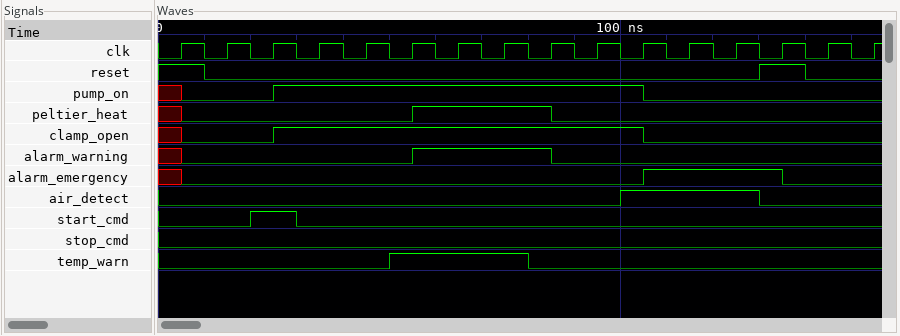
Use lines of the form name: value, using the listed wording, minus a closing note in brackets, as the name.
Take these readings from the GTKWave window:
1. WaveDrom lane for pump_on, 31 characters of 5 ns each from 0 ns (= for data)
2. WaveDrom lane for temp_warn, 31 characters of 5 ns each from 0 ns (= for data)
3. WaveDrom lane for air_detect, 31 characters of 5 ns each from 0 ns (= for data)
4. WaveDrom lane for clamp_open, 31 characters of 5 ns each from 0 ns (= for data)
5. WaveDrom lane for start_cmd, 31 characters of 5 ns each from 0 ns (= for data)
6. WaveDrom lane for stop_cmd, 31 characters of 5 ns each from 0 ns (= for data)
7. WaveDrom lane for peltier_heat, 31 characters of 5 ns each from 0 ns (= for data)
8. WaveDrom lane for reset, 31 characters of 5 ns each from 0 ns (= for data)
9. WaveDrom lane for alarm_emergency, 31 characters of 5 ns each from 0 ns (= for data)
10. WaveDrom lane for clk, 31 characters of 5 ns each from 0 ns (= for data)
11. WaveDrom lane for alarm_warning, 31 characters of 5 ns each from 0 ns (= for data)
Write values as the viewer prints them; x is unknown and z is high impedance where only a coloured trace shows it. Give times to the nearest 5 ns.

WaveDrom lane for pump_on, 31 characters of 5 ns each from 0 ns: {name: 'pump_on', wave: 'x0...1...............0.........'}
WaveDrom lane for temp_warn, 31 characters of 5 ns each from 0 ns: {name: 'temp_warn', wave: '0.........1.....0..............'}
WaveDrom lane for air_detect, 31 characters of 5 ns each from 0 ns: {name: 'air_detect', wave: '0...................1.....0....'}
WaveDrom lane for clamp_open, 31 characters of 5 ns each from 0 ns: {name: 'clamp_open', wave: 'x0...1...............0.........'}
WaveDrom lane for start_cmd, 31 characters of 5 ns each from 0 ns: {name: 'start_cmd', wave: '0...1.0........................'}
WaveDrom lane for stop_cmd, 31 characters of 5 ns each from 0 ns: {name: 'stop_cmd', wave: '0..............................'}
WaveDrom lane for peltier_heat, 31 characters of 5 ns each from 0 ns: {name: 'peltier_heat', wave: 'x0.........1.....0.............'}
WaveDrom lane for reset, 31 characters of 5 ns each from 0 ns: {name: 'reset', wave: '1.0.......................1.0..'}
WaveDrom lane for alarm_emergency, 31 characters of 5 ns each from 0 ns: {name: 'alarm_emergency', wave: 'x0...................1.....0...'}
WaveDrom lane for clk, 31 characters of 5 ns each from 0 ns: {name: 'clk', wave: '0101010101010101010101010101010'}
WaveDrom lane for alarm_warning, 31 characters of 5 ns each from 0 ns: {name: 'alarm_warning', wave: 'x0.........1.....0.............'}
